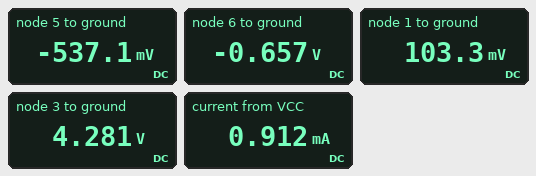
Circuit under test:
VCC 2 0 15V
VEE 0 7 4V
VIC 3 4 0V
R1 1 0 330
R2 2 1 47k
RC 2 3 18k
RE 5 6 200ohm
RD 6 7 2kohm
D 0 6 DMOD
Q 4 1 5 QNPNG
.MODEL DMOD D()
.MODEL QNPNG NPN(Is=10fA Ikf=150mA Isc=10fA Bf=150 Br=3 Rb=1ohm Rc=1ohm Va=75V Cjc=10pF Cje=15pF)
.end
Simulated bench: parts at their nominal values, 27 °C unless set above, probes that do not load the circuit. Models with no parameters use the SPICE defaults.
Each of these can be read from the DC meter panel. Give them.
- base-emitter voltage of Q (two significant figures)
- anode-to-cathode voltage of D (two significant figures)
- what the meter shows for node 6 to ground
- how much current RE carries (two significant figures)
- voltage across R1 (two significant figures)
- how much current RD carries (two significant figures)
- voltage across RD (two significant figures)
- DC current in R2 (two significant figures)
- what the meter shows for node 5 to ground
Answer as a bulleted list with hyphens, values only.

- 640 mV
- 660 mV
- -0.657 V
- 600 µA
- 100 mV
- 1.7 mA
- 3.3 V
- 320 µA
- -537.1 mV
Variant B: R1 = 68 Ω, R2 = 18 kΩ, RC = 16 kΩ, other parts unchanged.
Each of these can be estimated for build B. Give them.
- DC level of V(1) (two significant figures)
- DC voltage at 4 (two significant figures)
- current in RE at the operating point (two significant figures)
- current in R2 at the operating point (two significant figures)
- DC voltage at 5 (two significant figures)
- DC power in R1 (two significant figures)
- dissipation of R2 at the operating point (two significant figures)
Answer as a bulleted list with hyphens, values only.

- 56 mV
- 8.1 V
- 430 µA
- 830 µA
- -570 mV
- 47 µW
- 12 mW
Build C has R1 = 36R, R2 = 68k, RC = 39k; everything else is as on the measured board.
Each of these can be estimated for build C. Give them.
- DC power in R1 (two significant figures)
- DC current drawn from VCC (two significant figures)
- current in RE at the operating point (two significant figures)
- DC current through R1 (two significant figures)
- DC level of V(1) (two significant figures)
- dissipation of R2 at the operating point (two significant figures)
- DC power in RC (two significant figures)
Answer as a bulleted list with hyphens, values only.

- 1.7 µW
- 480 µA
- 260 µA
- 220 µA
- 7.9 mV
- 3.3 mW
- 2.7 mW
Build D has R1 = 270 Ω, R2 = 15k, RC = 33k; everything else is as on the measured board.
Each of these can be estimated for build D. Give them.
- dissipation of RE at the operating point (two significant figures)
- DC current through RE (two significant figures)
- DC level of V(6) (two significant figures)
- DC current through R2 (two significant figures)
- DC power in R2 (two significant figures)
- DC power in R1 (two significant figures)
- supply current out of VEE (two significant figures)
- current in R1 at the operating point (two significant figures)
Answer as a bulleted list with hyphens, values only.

- 130 µW
- 800 µA
- -650 mV
- 990 µA
- 15 mW
- 120 µW
- 1.7 mA
- 660 µA
